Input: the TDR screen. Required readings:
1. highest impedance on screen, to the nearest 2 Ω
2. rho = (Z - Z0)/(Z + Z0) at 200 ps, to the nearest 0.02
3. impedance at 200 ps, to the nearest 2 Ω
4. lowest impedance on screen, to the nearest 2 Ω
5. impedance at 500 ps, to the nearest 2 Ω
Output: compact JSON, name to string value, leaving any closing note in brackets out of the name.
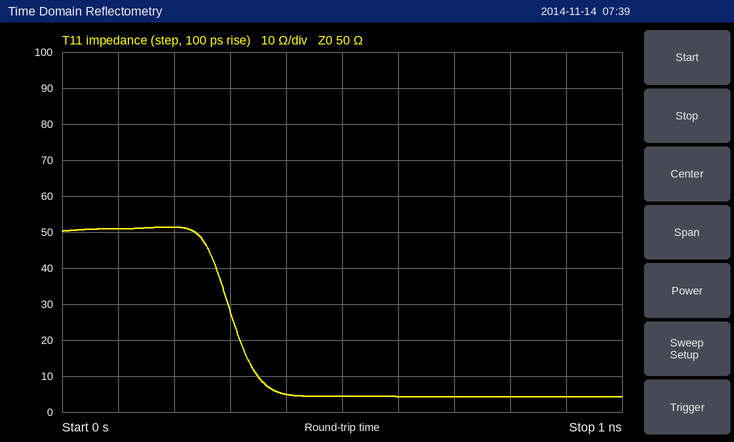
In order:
{"highest impedance on screen, to the nearest 2 Ω": "52 Ω", "rho = (Z - Z0)/(Z + Z0) at 200 ps, to the nearest 0.02": "+0.02", "impedance at 200 ps, to the nearest 2 Ω": "52 Ω", "lowest impedance on screen, to the nearest 2 Ω": "4 Ω", "impedance at 500 ps, to the nearest 2 Ω": "4 Ω"}
